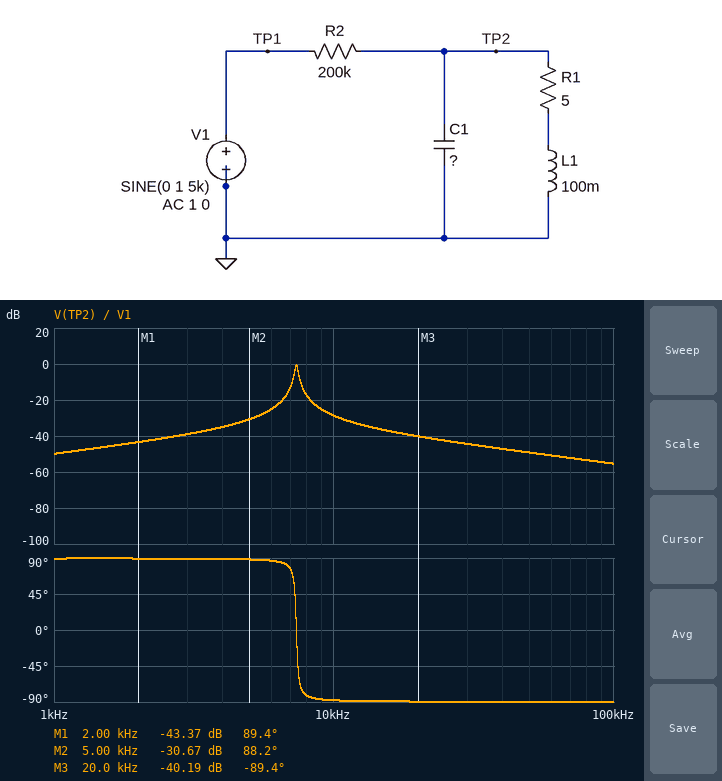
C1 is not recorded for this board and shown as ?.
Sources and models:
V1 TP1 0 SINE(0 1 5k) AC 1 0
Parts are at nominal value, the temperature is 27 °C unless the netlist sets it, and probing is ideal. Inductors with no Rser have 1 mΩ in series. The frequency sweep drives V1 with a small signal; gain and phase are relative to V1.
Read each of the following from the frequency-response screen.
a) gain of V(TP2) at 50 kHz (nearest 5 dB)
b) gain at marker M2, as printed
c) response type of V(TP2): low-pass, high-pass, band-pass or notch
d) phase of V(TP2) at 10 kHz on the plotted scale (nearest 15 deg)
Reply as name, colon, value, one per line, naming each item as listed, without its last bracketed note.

gain of V(TP2) at 50 kHz: -50 dB
gain at marker M2, as printed: -30.67 dB
response type of V(TP2): low-pass, high-pass, band-pass or notch: band-pass
phase of V(TP2) at 10 kHz on the plotted scale: -90 deg
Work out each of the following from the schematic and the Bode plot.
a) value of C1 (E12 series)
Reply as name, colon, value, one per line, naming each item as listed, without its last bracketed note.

value of C1: 4.7 nF
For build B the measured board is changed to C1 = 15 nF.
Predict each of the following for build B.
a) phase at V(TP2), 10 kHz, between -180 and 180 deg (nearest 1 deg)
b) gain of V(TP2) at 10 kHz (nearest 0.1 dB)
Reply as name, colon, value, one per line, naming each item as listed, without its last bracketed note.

phase at V(TP2), 10 kHz, between -180 and 180 deg: -90 deg
gain of V(TP2) at 10 kHz: -43.9 dB
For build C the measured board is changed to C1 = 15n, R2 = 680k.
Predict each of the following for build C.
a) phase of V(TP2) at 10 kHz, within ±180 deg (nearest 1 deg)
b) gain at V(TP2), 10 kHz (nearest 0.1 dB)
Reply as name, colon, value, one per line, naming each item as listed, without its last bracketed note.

phase of V(TP2) at 10 kHz, within ±180 deg: -90 deg
gain at V(TP2), 10 kHz: -54.5 dB
